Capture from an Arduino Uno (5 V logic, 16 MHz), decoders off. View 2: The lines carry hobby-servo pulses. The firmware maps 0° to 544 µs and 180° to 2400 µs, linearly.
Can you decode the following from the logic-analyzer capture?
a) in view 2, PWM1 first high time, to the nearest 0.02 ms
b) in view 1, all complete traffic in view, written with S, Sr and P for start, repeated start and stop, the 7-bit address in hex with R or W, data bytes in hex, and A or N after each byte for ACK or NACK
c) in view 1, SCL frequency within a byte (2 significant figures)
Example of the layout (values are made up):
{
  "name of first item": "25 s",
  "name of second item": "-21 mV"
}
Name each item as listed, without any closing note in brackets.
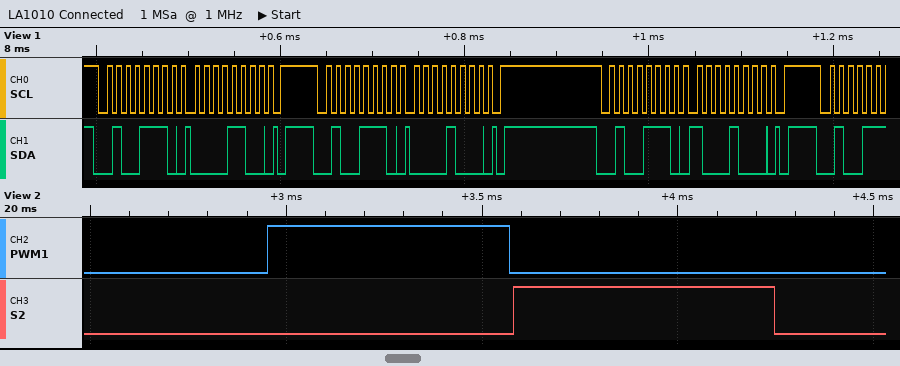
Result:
{
  "in view 2, PWM1 first high time, to the nearest 0.02 ms": "0.62 ms",
  "in view 1, all complete traffic in view, written with S, Sr and P for start, repeated start and stop, the 7-bit address in hex with R or W, data bytes in hex, and A or N after each byte for ACK or NACK": "S 27W A 0C A P S 27W A 08 A P S 27W A 88 A P",
  "in view 1, SCL frequency within a byte": "100 kHz"
}
